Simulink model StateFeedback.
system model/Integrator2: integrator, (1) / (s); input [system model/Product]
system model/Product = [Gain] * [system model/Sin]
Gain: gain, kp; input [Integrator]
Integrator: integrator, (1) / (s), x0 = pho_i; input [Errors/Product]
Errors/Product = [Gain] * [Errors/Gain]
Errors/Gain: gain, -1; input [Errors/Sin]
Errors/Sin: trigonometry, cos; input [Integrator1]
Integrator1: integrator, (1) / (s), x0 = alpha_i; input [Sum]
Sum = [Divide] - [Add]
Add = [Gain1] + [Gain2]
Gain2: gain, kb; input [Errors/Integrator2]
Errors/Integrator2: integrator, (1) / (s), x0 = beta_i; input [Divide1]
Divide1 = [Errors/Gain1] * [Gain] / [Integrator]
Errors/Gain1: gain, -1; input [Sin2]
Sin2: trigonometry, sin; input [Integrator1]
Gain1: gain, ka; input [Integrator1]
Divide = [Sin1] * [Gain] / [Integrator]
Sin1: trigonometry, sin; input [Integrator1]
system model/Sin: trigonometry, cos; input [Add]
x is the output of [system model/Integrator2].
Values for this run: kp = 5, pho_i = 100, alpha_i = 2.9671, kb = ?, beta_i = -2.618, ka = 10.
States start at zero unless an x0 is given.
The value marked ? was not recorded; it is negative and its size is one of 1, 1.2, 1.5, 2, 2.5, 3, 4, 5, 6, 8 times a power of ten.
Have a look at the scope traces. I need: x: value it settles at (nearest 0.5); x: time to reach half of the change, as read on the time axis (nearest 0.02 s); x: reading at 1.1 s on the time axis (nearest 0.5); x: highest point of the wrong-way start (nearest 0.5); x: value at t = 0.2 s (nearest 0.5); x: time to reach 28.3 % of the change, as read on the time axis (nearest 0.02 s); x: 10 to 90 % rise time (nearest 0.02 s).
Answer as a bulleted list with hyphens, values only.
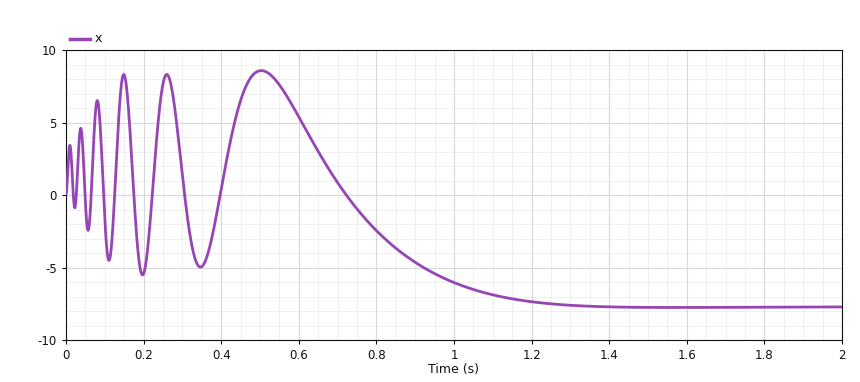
- -7.5
- 0.10 s
- -7.0
- 8.5
- -5.5
- 0.06 s
- 1.08 s
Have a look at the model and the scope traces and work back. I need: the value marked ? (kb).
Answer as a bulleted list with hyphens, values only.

- -1.2
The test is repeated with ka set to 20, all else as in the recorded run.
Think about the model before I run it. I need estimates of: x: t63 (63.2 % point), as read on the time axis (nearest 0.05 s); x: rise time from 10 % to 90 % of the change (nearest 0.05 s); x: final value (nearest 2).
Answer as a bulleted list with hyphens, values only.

- 0.40 s
- 0.55 s
- 28
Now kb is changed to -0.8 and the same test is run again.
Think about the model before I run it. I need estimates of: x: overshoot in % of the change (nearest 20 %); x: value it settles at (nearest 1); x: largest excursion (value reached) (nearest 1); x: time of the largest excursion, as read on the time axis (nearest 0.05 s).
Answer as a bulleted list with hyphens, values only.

- 120 %
- 4
- 9
- 0.25 s
